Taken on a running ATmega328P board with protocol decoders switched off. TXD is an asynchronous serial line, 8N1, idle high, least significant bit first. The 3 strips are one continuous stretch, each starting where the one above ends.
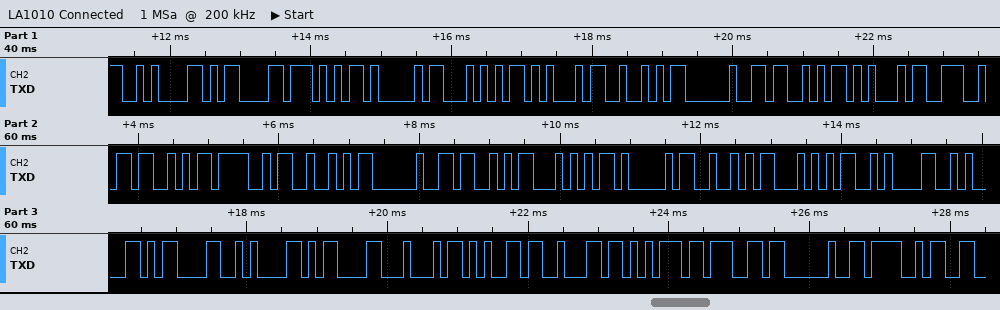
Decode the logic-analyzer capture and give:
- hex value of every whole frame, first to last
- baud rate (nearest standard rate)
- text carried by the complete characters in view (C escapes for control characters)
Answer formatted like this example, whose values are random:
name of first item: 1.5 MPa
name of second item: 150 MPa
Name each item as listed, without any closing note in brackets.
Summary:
hex value of every whole frame, first to last: 0x0A 0x0D 0x57 0x41 0x54 0x45 0x52 0x20 0x53 0x45 0x4E 0x53 0x4F 0x52 0x20 0x53 0x54 0x41 0x52 0x54 0x0A 0x0A 0x0D 0x0A 0x0D 0x44 0x65 0x62 0x75 0x67 0x20 0x4F
baud rate: 9600 baud
text carried by the complete characters in view: "\n\rWATER SENSOR START\n\n\r\n\rDebug O"
